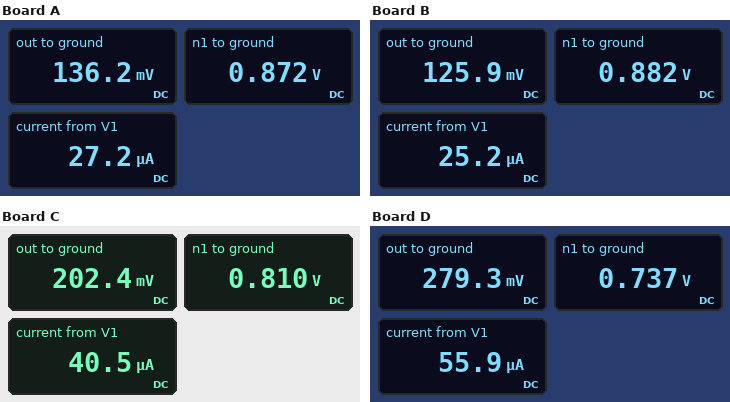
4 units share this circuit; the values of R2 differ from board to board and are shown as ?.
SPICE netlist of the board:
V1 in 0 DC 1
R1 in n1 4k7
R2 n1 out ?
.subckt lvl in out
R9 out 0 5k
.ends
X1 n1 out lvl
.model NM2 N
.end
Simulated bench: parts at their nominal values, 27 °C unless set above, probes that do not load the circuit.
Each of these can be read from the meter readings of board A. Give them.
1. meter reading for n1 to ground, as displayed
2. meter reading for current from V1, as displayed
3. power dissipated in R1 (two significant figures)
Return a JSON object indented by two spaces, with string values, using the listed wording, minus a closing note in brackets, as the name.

{
  "meter reading for n1 to ground, as displayed": "0.872 V",
  "meter reading for current from V1, as displayed": "27.2 µA",
  "power dissipated in R1": "3.5 µW"
}
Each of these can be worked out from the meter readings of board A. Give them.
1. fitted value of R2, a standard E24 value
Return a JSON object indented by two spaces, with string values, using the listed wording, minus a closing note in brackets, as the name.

{
  "fitted value of R2, a standard E24 value": "27 kΩ"
}
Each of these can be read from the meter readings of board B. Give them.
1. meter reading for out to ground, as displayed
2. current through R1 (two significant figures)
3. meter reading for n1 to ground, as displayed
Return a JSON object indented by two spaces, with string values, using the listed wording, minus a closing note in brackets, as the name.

{
  "meter reading for out to ground, as displayed": "125.9 mV",
  "current through R1": "25 µA",
  "meter reading for n1 to ground, as displayed": "0.882 V"
}
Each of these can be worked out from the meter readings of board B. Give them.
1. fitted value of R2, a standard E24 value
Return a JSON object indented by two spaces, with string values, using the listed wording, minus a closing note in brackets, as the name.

{
  "fitted value of R2, a standard E24 value": "30 kΩ"
}
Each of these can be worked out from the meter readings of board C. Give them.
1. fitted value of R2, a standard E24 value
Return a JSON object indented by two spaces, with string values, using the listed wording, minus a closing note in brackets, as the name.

{
  "fitted value of R2, a standard E24 value": "15 kΩ"
}
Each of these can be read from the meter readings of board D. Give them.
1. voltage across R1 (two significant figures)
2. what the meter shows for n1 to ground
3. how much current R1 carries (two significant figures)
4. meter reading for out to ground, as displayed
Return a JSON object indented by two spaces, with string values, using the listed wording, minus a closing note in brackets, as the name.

{
  "voltage across R1": "260 mV",
  "what the meter shows for n1 to ground": "0.737 V",
  "how much current R1 carries": "56 µA",
  "meter reading for out to ground, as displayed": "279.3 mV"
}
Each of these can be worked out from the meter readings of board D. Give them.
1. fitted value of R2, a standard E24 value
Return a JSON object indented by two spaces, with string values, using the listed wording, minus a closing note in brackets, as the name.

{
  "fitted value of R2, a standard E24 value": "8.2 kΩ"
}
